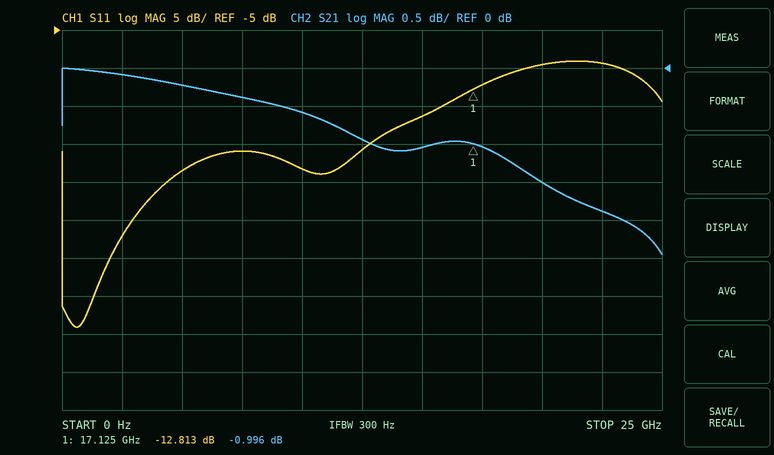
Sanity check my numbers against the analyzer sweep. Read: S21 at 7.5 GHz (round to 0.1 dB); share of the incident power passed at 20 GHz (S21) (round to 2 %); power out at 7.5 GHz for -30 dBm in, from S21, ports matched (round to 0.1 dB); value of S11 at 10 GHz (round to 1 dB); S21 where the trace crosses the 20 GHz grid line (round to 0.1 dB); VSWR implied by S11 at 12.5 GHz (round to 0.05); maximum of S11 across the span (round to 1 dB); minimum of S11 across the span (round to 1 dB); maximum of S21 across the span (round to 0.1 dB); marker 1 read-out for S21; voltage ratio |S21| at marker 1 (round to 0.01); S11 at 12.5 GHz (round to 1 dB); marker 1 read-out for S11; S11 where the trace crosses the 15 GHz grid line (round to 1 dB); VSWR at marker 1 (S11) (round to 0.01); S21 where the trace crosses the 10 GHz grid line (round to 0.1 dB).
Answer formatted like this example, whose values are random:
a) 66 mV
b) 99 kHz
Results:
a) -0.4 dB
b) 70 %
c) -30.4 dBm
d) -23 dB
e) -1.5 dB
f) 1.20
g) -9 dB
h) -44 dB
i) 0.0 dB
j) -0.996 dB
k) 0.89
l) -21 dB
m) -12.813 dB
n) -16 dB
o) 1.59
p) -0.6 dB
